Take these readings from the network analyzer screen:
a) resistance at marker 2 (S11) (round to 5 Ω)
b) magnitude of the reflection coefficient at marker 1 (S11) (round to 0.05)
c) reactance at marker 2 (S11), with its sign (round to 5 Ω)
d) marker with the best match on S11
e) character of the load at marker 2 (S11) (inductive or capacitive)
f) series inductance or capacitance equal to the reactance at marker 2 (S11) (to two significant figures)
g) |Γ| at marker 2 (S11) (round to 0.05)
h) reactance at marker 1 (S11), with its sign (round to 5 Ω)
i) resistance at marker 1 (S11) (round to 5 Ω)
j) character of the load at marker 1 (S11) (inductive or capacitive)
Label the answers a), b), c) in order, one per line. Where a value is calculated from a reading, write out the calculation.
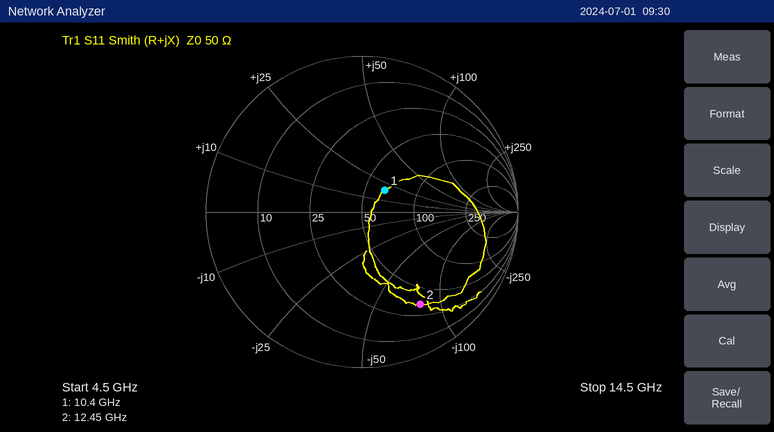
a) 35 Ω
b) 0.20
c) -80 Ω
d) marker 1
e) capacitive
f) C = 1/(2π × 12.45 GHz × 80 Ω) ≈ 160 fF
g) 0.70
h) +20 Ω
i) 65 Ω
j) inductive
